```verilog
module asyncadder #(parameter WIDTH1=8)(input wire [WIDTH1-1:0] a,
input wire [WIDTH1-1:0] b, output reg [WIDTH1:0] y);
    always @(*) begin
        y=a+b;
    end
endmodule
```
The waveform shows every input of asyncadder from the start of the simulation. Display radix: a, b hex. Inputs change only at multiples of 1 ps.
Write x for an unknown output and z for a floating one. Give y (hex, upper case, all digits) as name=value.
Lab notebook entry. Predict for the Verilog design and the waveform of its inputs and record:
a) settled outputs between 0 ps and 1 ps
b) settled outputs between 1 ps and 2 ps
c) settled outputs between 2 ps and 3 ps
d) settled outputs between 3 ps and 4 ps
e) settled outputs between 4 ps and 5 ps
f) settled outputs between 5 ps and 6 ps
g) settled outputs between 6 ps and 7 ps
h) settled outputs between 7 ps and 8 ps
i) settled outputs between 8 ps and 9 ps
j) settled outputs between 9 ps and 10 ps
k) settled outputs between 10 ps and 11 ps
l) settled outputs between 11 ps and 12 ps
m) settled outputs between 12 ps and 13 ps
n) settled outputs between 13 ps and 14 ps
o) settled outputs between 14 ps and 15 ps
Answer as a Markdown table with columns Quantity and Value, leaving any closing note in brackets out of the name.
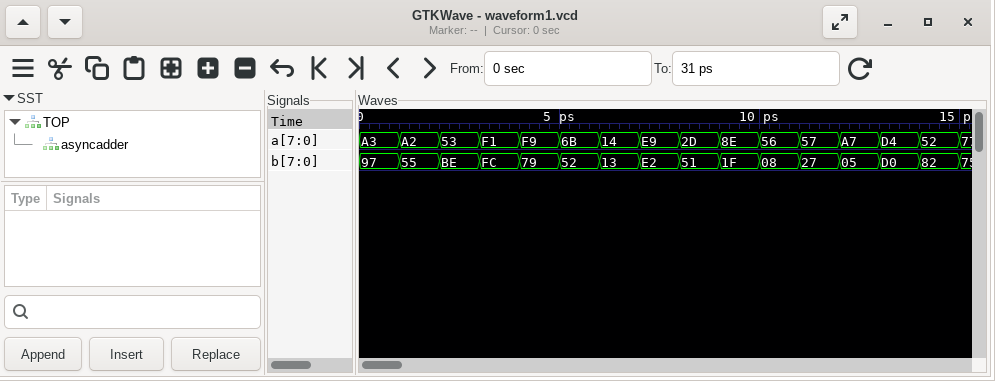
| Quantity | Value |
|---|---|
| settled outputs between 0 ps and 1 ps | y=13A |
| settled outputs between 1 ps and 2 ps | y=0F7 |
| settled outputs between 2 ps and 3 ps | y=111 |
| settled outputs between 3 ps and 4 ps | y=1ED |
| settled outputs between 4 ps and 5 ps | y=172 |
| settled outputs between 5 ps and 6 ps | y=0BD |
| settled outputs between 6 ps and 7 ps | y=027 |
| settled outputs between 7 ps and 8 ps | y=1CB |
| settled outputs between 8 ps and 9 ps | y=07E |
| settled outputs between 9 ps and 10 ps | y=0AD |
| settled outputs between 10 ps and 11 ps | y=05E |
| settled outputs between 11 ps and 12 ps | y=07E |
| settled outputs between 12 ps and 13 ps | y=0AC |
| settled outputs between 13 ps and 14 ps | y=1A4 |
| settled outputs between 14 ps and 15 ps | y=0D4 |
